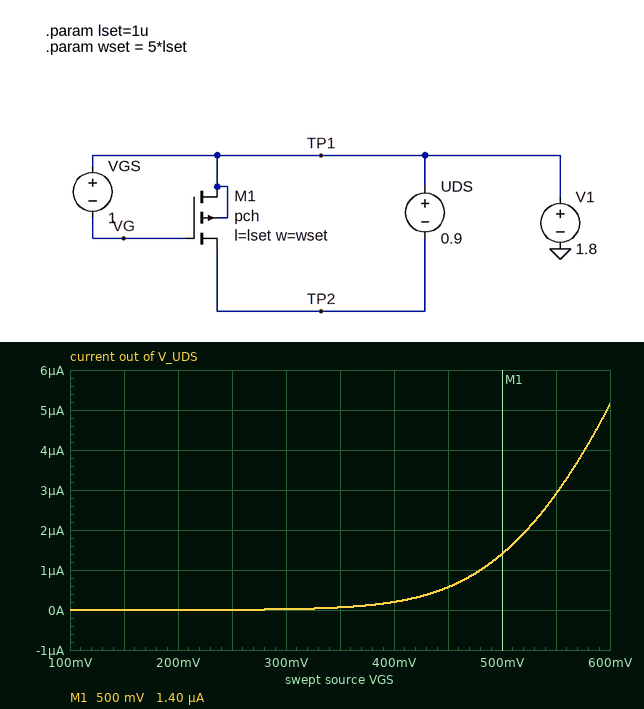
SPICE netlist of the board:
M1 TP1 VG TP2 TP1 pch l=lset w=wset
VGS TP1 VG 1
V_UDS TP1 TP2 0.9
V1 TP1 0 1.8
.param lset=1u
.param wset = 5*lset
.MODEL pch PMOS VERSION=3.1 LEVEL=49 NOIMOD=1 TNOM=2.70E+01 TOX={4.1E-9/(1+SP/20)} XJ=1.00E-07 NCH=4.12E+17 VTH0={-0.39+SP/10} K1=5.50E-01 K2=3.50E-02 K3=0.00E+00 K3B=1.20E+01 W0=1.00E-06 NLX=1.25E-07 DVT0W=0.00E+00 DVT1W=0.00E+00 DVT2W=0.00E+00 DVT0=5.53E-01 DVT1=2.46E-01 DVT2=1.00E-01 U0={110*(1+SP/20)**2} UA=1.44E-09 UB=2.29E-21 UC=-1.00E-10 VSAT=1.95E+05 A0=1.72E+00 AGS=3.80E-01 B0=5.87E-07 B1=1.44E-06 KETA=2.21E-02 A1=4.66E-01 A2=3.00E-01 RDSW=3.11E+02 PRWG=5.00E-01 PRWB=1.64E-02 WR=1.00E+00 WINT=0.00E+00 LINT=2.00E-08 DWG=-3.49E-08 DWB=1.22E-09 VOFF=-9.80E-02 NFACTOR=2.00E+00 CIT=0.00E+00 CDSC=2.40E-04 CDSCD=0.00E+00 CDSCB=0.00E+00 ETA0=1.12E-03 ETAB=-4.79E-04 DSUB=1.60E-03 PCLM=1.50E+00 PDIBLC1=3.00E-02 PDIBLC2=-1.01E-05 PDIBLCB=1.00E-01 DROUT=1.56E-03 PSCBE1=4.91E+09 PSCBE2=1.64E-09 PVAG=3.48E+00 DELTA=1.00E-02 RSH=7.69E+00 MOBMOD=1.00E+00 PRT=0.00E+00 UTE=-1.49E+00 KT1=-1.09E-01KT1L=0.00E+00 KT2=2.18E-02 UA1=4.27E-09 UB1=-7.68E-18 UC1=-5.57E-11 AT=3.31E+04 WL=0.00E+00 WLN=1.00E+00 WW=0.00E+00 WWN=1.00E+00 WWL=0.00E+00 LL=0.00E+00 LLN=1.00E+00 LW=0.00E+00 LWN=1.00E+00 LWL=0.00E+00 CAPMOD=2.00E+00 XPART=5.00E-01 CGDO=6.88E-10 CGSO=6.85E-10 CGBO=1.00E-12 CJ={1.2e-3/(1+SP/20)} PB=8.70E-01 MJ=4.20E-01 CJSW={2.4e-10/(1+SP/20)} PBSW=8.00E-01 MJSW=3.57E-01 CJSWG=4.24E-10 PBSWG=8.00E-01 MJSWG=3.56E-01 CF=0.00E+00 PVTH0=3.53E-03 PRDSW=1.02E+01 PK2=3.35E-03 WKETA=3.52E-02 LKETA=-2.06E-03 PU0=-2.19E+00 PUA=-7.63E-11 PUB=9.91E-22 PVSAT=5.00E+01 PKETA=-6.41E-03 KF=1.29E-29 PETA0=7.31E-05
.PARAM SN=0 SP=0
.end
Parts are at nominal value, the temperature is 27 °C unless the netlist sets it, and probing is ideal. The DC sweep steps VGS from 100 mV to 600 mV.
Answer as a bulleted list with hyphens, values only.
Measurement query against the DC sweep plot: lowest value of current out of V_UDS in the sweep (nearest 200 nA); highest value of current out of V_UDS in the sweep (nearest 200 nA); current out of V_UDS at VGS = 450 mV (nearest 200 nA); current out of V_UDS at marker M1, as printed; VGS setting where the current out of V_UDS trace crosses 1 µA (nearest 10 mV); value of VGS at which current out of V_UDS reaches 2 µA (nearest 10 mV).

- 0 A
- 5.2 µA
- 600 nA
- 1.40 µA
- 480 mV
- 520 mV
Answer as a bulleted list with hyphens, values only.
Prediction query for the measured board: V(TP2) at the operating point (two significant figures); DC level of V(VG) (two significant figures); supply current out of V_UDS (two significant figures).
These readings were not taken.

- 900 mV
- 800 mV
- 43 µA
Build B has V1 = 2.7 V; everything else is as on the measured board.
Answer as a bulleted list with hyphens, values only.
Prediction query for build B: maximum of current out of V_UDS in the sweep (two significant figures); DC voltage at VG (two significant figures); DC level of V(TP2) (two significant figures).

- 5.1 µA
- 1.7 V
- 1.8 V
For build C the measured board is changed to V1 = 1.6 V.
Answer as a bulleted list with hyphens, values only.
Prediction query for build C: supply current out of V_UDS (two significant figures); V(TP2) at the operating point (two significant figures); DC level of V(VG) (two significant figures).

- 43 µA
- 700 mV
- 600 mV
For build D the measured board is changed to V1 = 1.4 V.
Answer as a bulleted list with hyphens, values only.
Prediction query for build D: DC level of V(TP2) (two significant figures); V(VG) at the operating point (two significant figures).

- 500 mV
- 400 mV
